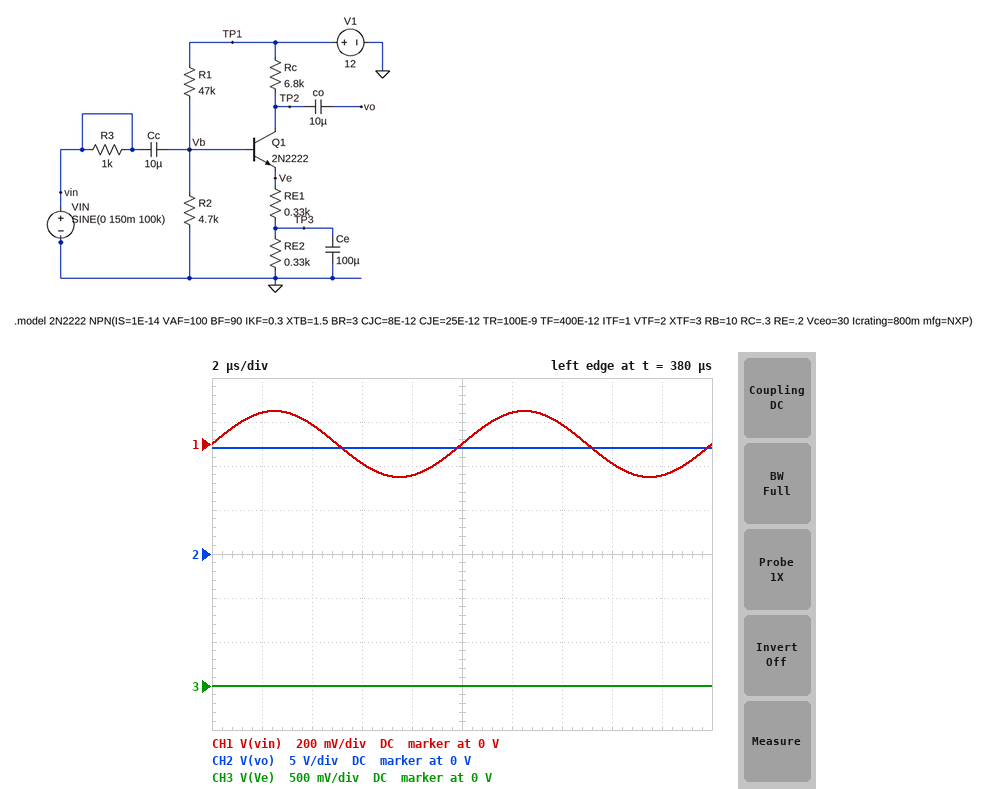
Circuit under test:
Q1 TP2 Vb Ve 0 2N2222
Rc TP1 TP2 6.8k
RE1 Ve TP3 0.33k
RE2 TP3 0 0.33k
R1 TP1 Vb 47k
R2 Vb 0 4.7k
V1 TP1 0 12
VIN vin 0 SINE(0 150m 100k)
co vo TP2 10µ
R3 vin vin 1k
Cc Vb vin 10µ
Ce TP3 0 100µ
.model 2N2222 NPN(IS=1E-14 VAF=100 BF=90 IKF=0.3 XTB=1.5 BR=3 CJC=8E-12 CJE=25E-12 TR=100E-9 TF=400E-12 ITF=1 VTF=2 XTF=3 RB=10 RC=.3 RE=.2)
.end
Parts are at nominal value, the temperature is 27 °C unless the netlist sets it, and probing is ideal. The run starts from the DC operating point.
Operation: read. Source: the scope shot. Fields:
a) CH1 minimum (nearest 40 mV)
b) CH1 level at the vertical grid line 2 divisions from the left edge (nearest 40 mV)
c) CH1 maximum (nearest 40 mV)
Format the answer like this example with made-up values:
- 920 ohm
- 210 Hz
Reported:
- -160 mV
- 80 mV
- 160 mV
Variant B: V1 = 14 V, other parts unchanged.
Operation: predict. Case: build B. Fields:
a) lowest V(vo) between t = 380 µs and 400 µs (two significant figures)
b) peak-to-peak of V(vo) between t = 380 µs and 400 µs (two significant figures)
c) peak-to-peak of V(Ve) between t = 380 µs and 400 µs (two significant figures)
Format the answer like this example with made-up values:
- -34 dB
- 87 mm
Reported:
- 14 V
- 3.8 mV
- 1.6 mV
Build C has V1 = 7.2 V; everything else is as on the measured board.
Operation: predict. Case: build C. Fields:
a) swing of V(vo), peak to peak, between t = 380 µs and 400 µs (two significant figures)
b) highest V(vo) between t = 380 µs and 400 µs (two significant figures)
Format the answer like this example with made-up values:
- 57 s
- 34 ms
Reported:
- 4.7 mV
- 7.2 V
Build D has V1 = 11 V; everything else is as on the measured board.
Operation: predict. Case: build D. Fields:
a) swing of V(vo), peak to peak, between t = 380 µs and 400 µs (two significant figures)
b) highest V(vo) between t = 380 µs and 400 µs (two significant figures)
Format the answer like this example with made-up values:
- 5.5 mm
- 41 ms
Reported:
- 4.1 mV
- 11 V
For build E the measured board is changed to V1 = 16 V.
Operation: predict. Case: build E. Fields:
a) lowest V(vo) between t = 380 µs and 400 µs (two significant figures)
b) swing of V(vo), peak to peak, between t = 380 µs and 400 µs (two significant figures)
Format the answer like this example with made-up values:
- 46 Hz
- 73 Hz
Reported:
- 16 V
- 3.7 mV
